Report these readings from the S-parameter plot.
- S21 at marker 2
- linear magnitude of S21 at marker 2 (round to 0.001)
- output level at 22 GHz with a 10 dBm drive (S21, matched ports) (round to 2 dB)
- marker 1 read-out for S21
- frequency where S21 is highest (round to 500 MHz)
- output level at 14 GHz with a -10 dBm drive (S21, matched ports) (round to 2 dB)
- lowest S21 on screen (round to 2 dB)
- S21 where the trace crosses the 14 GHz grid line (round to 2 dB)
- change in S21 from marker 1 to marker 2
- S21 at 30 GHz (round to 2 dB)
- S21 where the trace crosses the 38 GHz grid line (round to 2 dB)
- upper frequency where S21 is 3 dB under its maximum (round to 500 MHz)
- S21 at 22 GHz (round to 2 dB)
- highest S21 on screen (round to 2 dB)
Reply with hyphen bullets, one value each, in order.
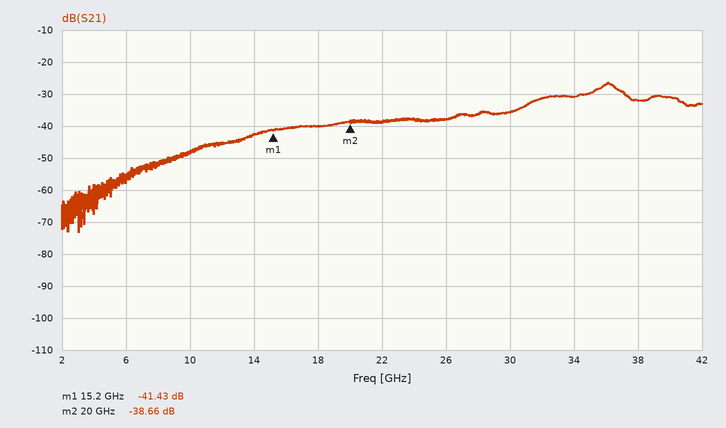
- -38.66 dB
- 0.012
- -28 dBm
- -41.43 dB
- 36.0 GHz
- -52 dBm
- -74 dB
- -42 dB
- 2.77 dB
- -36 dB
- -32 dB
- 37.0 GHz
- -38 dB
- -26 dB
